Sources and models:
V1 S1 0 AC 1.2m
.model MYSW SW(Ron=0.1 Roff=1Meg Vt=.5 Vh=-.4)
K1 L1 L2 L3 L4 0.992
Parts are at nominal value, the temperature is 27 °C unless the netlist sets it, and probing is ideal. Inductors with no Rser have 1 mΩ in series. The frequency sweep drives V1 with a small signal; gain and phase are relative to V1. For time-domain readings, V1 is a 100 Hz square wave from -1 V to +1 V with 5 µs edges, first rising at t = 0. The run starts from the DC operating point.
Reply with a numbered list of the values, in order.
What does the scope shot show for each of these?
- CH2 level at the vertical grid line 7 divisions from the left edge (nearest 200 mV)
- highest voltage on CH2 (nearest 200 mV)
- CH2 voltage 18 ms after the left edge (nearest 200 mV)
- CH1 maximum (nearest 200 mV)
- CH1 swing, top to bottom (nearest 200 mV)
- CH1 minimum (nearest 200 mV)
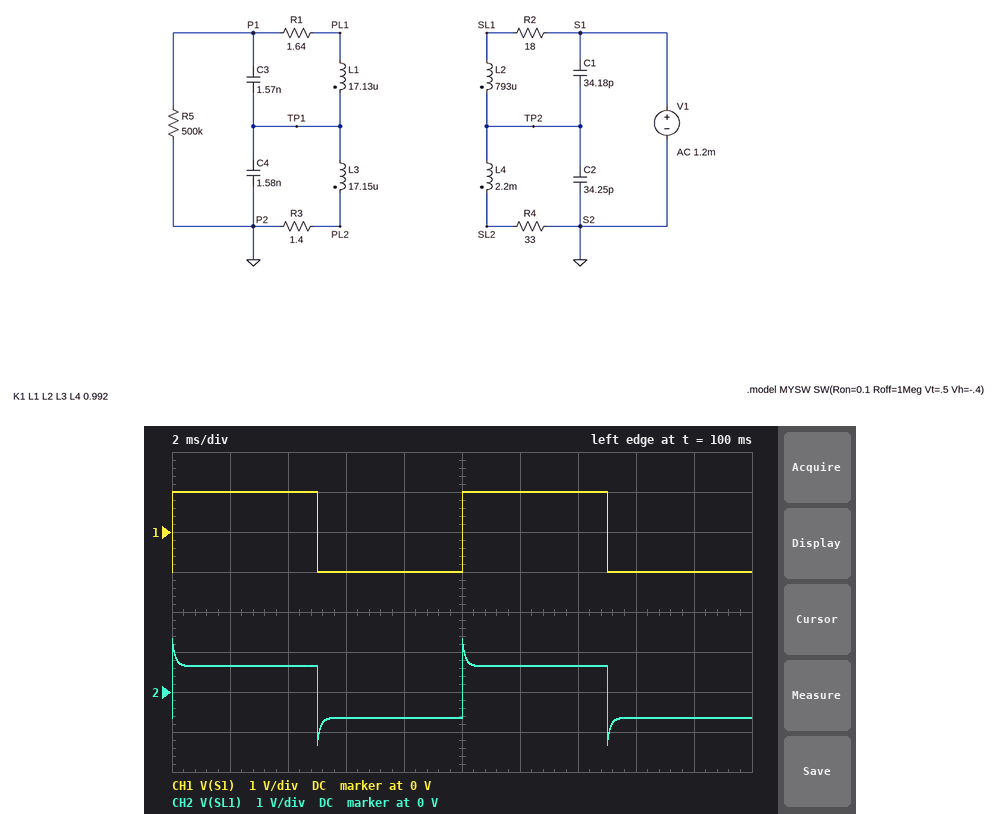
1. 600 mV
2. 1.4 V
3. -600 mV
4. 1.0 V
5. 2.0 V
6. -1.0 V
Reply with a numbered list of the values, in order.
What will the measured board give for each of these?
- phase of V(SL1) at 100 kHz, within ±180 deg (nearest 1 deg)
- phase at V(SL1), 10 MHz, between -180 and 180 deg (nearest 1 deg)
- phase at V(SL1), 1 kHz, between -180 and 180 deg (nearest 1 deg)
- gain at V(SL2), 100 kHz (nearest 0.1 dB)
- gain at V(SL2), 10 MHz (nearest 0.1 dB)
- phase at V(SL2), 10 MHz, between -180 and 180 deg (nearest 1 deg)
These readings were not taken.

1. 0 deg
2. 4 deg
3. 12 deg
4. -40.7 dB
5. -40.6 dB
6. 112 deg
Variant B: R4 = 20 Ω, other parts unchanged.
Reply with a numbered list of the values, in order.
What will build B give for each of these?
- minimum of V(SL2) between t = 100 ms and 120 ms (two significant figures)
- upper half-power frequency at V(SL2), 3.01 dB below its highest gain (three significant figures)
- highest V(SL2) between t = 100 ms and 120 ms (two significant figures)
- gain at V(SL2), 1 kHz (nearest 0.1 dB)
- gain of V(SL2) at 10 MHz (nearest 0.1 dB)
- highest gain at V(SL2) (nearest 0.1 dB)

1. -530 mV
2. 1.08 kHz
3. 530 mV
4. -8.3 dB
5. -44.9 dB
6. -5.6 dB
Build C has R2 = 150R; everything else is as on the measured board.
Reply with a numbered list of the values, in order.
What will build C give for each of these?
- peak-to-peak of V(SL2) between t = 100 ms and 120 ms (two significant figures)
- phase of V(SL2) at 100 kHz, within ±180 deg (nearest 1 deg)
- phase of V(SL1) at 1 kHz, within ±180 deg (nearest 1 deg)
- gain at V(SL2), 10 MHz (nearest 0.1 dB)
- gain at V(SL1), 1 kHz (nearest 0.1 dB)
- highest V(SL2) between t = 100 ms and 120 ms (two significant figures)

1. 360 mV
2. -87 deg
3. 36 deg
4. -36.6 dB
5. -11.7 dB
6. 180 mV
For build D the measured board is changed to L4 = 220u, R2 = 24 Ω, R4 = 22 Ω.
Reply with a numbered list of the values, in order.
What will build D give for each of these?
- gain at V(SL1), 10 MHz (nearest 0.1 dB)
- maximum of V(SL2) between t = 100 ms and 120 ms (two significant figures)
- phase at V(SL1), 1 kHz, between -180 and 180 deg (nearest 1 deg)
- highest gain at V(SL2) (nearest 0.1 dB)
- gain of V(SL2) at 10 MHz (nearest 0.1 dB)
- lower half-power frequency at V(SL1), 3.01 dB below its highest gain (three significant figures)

1. -0.1 dB
2. 480 mV
3. 14 deg
4. -6.4 dB
5. -36.2 dB
6. 3.92 kHz
